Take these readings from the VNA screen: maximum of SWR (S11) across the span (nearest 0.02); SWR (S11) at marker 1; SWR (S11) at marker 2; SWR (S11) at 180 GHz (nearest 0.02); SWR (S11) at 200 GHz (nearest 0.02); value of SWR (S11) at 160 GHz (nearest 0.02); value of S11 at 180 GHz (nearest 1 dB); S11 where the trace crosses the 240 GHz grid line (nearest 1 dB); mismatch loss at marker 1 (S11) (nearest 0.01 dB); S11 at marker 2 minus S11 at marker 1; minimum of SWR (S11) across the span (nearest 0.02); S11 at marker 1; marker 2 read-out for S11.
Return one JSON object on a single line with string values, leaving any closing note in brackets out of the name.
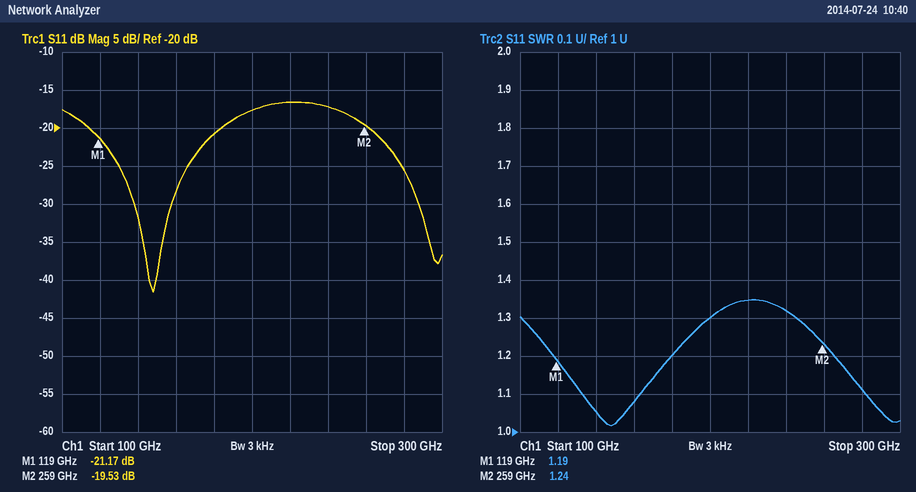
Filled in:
{"maximum of SWR (S11) across the span": "1.34", "SWR (S11) at marker 1": "1.19", "SWR (S11) at marker 2": "1.24", "SWR (S11) at 180 GHz": "1.20", "SWR (S11) at 200 GHz": "1.30", "value of SWR (S11) at 160 GHz": "1.08", "value of S11 at 180 GHz": "-21 dB", "S11 where the trace crosses the 240 GHz grid line": "-17 dB", "mismatch loss at marker 1 (S11)": "0.03 dB", "S11 at marker 2 minus S11 at marker 1": "1.64 dB", "minimum of SWR (S11) across the span": "1.02", "S11 at marker 1": "-21.17 dB", "marker 2 read-out for S11": "-19.53 dB"}
